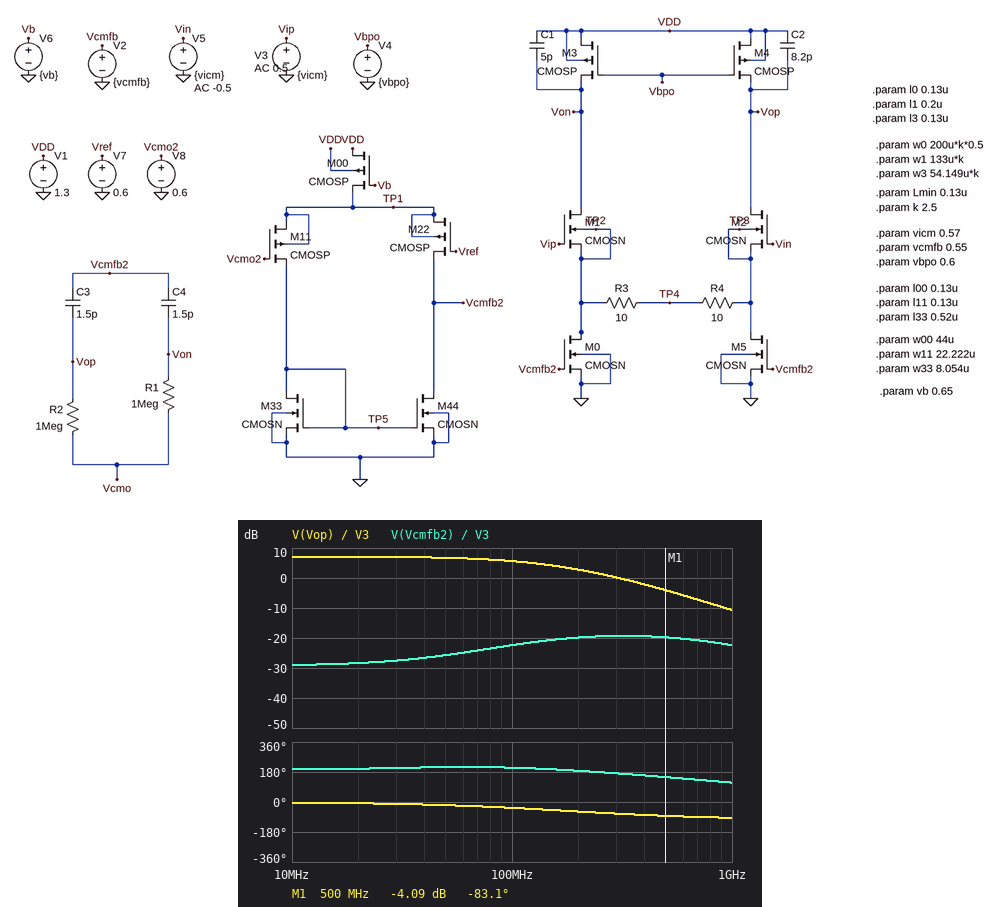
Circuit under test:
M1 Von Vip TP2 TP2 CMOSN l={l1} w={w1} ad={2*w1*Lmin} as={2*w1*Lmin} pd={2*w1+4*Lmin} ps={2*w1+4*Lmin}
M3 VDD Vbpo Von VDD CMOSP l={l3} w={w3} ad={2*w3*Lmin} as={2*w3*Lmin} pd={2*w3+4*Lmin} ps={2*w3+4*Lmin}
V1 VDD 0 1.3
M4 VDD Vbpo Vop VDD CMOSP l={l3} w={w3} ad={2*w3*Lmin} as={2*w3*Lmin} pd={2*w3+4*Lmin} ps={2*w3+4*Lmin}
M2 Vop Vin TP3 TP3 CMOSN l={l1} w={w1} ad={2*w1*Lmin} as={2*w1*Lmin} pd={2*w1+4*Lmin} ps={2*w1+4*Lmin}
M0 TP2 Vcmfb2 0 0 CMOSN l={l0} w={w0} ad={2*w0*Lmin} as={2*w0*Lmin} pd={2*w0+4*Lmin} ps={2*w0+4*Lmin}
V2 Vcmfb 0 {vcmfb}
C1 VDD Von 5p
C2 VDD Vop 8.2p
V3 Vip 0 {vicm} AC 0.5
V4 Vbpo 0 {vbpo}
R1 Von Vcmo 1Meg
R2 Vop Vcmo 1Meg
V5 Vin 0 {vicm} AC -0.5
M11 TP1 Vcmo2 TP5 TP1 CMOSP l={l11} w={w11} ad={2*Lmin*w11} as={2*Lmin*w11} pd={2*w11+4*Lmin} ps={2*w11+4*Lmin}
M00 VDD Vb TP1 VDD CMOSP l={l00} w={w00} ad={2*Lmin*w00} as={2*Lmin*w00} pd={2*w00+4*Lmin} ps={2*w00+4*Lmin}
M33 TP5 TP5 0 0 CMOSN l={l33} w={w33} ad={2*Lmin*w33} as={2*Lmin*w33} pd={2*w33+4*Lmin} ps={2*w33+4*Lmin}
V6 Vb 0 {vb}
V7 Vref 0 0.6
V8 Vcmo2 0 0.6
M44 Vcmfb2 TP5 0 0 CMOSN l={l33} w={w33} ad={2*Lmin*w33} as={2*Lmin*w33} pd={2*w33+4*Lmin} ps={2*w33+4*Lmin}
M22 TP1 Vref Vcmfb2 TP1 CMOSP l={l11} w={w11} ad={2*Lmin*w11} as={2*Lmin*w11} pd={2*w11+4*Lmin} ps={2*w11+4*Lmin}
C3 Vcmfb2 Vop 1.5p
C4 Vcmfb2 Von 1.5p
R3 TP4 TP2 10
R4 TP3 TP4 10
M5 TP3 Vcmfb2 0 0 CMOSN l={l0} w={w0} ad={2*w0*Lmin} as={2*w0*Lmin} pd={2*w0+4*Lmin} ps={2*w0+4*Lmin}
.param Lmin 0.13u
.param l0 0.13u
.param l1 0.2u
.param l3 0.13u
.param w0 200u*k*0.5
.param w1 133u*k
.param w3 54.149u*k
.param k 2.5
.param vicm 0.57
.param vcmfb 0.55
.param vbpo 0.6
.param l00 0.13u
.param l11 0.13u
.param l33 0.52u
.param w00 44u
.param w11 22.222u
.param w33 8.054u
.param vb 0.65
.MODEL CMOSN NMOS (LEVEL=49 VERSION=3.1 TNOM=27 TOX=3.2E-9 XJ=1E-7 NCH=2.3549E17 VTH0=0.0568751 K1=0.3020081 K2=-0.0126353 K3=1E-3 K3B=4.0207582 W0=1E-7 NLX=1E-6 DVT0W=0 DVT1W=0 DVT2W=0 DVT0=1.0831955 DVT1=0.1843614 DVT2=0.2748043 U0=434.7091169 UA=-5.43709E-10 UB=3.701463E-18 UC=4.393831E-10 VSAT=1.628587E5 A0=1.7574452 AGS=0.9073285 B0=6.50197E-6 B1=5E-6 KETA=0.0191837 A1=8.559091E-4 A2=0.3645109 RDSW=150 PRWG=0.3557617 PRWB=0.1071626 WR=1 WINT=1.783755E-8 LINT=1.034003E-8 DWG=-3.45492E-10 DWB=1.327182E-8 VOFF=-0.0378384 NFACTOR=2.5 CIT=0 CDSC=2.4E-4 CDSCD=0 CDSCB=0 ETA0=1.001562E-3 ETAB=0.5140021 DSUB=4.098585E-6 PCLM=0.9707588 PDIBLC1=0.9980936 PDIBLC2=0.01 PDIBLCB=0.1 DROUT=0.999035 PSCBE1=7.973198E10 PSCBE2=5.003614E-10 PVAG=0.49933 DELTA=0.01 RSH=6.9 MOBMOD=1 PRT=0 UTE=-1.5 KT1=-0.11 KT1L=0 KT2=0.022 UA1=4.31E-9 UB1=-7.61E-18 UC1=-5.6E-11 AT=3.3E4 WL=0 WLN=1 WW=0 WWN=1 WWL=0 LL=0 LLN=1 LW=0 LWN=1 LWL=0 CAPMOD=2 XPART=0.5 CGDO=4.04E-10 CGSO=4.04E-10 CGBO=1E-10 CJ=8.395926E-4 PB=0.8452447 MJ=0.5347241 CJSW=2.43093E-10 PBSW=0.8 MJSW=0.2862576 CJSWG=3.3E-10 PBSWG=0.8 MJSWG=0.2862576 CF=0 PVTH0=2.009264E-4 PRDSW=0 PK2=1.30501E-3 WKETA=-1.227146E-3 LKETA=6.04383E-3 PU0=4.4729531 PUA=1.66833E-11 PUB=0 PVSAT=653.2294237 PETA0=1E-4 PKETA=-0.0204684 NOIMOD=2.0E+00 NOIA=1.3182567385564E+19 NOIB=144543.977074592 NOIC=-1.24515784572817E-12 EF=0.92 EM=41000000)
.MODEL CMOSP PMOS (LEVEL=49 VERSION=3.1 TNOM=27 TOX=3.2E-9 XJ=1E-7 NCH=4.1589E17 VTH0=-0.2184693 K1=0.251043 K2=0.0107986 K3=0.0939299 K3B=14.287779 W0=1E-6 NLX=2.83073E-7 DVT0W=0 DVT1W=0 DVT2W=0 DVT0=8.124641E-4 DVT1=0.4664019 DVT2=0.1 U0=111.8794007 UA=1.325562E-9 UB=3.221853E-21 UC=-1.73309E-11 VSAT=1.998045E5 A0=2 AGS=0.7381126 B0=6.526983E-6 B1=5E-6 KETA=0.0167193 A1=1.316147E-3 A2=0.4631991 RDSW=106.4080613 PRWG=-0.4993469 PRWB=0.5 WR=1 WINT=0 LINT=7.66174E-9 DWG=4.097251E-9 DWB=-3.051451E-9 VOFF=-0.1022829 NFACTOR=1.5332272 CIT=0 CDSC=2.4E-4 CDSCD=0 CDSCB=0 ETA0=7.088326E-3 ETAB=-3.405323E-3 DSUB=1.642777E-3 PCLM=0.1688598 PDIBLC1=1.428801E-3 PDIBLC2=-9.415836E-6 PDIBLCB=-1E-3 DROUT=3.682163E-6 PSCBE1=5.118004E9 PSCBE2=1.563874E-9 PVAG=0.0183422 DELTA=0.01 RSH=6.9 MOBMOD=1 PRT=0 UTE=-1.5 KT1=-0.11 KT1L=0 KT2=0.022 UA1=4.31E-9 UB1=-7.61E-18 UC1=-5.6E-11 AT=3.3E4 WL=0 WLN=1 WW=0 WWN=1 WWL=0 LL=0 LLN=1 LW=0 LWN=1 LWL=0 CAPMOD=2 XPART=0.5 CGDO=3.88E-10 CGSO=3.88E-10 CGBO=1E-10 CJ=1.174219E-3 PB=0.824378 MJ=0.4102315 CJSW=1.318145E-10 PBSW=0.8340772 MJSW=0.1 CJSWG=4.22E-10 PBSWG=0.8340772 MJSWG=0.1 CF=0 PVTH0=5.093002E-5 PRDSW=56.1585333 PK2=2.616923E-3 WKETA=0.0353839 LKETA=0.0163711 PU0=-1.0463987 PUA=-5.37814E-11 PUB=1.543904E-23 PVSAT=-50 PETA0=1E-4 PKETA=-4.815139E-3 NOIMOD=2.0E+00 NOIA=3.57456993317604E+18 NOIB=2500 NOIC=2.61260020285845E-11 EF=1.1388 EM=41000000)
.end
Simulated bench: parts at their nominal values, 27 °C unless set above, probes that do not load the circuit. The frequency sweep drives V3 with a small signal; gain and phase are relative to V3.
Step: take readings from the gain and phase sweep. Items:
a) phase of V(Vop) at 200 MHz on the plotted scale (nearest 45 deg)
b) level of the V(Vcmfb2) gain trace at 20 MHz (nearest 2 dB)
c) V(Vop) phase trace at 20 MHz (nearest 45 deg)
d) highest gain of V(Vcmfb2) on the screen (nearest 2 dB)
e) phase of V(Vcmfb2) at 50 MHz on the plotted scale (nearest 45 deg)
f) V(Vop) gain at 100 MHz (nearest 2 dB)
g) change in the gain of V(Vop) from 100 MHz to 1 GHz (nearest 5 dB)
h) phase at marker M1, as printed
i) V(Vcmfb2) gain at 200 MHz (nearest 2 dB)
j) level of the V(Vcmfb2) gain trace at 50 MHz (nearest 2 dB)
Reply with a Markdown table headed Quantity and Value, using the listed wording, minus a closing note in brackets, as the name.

| Quantity | Value |
|---|---|
| phase of V(Vop) at 200 MHz on the plotted scale | -45 deg |
| level of the V(Vcmfb2) gain trace at 20 MHz | -28 dB |
| V(Vop) phase trace at 20 MHz | 0 deg |
| highest gain of V(Vcmfb2) on the screen | -20 dB |
| phase of V(Vcmfb2) at 50 MHz on the plotted scale | 225 deg |
| V(Vop) gain at 100 MHz | 6 dB |
| change in the gain of V(Vop) from 100 MHz to 1 GHz | -15 dB |
| phase at marker M1, as printed | -83.1 deg |
| V(Vcmfb2) gain at 200 MHz | -20 dB |
| level of the V(Vcmfb2) gain trace at 50 MHz | -26 dB |
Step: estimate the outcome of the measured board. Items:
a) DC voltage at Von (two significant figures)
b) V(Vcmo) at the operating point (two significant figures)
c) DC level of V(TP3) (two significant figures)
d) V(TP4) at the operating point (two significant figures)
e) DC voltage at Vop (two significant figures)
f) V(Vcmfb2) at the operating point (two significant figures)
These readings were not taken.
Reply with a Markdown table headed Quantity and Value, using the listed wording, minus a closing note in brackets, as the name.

| Quantity | Value |
|---|---|
| DC voltage at Von | 1.1 V |
| V(Vcmo) at the operating point | 1.1 V |
| DC level of V(TP3) | 130 mV |
| V(TP4) at the operating point | 130 mV |
| DC voltage at Vop | 1.1 V |
| V(Vcmfb2) at the operating point | 550 mV |
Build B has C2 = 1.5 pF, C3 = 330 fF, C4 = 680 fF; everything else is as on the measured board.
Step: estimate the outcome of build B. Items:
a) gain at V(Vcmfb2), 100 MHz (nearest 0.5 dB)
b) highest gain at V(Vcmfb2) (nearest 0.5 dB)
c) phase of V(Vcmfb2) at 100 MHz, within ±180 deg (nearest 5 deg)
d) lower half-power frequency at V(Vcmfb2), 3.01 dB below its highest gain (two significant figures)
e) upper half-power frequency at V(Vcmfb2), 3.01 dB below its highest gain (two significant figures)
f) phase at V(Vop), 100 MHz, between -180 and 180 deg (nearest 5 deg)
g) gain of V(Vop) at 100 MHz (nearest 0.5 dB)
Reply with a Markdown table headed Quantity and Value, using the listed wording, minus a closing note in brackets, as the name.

| Quantity | Value |
|---|---|
| gain at V(Vcmfb2), 100 MHz | -15.5 dB |
| highest gain at V(Vcmfb2) | -15.0 dB |
| phase of V(Vcmfb2) at 100 MHz, within ±180 deg | 155 deg |
| lower half-power frequency at V(Vcmfb2), 3.01 dB below its highest gain | 2.8 MHz |
| upper half-power frequency at V(Vcmfb2), 3.01 dB below its highest gain | 380 MHz |
| phase at V(Vop), 100 MHz, between -180 and 180 deg | -15 deg |
| gain of V(Vop) at 100 MHz | 8.5 dB |
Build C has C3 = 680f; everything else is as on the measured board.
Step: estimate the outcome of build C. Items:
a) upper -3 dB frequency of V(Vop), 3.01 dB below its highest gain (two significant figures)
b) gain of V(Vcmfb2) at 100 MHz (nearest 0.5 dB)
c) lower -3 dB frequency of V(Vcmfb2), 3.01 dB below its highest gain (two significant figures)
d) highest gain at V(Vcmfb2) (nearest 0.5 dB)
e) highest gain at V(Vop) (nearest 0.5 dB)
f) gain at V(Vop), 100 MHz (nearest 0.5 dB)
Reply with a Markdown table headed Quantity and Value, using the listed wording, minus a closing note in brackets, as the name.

| Quantity | Value |
|---|---|
| upper -3 dB frequency of V(Vop), 3.01 dB below its highest gain | 150 MHz |
| gain of V(Vcmfb2) at 100 MHz | -12.5 dB |
| lower -3 dB frequency of V(Vcmfb2), 3.01 dB below its highest gain | 2.1 MHz |
| highest gain at V(Vcmfb2) | -12.0 dB |
| highest gain at V(Vop) | 9.0 dB |
| gain at V(Vop), 100 MHz | 7.5 dB |
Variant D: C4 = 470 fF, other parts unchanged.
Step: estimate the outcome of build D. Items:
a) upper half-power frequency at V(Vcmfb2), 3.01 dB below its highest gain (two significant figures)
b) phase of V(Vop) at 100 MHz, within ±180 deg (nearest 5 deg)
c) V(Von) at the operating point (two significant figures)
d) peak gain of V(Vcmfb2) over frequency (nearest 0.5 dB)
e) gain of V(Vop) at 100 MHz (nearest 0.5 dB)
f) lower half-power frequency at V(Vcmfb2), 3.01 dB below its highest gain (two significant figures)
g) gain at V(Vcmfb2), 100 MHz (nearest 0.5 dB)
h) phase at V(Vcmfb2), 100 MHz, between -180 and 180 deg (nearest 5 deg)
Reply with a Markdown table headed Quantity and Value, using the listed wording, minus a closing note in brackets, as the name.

| Quantity | Value |
|---|---|
| upper half-power frequency at V(Vcmfb2), 3.01 dB below its highest gain | 220 MHz |
| phase of V(Vop) at 100 MHz, within ±180 deg | -30 deg |
| V(Von) at the operating point | 1.1 V |
| peak gain of V(Vcmfb2) over frequency | -13.0 dB |
| gain of V(Vop) at 100 MHz | 2.0 dB |
| lower half-power frequency at V(Vcmfb2), 3.01 dB below its highest gain | 1.6 MHz |
| gain at V(Vcmfb2), 100 MHz | -14.0 dB |
| phase at V(Vcmfb2), 100 MHz, between -180 and 180 deg | -20 deg |
